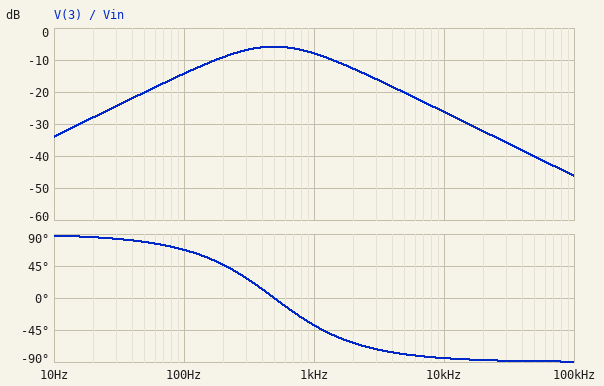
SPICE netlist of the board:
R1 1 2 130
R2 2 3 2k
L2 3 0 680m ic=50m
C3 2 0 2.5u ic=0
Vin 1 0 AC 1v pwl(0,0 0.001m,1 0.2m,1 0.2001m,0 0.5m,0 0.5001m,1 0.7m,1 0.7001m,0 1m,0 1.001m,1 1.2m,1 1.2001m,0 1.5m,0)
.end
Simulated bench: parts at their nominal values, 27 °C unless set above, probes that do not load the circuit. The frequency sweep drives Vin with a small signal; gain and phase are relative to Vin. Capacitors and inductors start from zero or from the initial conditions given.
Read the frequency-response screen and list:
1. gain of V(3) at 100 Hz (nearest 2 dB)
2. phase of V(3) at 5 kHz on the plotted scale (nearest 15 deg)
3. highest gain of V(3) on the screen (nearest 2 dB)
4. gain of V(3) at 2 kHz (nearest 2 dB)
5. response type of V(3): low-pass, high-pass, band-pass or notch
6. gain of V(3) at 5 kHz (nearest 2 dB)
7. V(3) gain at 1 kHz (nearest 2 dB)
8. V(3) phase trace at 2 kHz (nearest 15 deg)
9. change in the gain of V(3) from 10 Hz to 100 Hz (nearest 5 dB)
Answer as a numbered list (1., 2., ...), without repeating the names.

1. -14 dB
2. -75 deg
3. -6 dB
4. -12 dB
5. band-pass
6. -20 dB
7. -8 dB
8. -60 deg
9. 20 dB
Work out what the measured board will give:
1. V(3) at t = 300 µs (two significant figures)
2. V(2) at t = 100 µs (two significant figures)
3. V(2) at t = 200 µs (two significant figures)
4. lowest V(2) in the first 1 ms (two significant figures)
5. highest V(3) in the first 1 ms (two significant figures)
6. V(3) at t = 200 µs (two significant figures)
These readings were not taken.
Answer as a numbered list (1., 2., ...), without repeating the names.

1. -43 V
2. -1.2 V
3. -1.7 V
4. -2.1 V
5. -4.9 V
6. -57 V
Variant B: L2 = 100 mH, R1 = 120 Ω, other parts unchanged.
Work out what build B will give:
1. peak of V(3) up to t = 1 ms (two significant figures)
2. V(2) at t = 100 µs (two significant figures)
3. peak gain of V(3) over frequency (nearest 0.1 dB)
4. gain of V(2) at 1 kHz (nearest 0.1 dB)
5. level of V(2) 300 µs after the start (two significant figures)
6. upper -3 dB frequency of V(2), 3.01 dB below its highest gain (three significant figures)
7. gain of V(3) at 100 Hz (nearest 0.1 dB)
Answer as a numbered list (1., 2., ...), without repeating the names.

1. 120 mV
2. -410 mV
3. -16.9 dB
4. -6.6 dB
5. -82 mV
6. 569 Hz
7. -30.7 dB
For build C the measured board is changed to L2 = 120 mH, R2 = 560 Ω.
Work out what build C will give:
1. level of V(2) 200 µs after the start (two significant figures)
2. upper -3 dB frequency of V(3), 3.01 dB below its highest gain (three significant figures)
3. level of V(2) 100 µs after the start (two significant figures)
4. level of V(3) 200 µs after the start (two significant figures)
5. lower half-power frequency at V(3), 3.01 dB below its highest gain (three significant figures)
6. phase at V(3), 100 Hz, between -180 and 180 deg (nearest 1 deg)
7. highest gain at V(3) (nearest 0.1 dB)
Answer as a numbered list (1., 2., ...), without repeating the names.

1. -1.4 V
2. 1.53 kHz
3. -1.1 V
4. -12 V
5. 294 Hz
6. 74 deg
7. -8.0 dB
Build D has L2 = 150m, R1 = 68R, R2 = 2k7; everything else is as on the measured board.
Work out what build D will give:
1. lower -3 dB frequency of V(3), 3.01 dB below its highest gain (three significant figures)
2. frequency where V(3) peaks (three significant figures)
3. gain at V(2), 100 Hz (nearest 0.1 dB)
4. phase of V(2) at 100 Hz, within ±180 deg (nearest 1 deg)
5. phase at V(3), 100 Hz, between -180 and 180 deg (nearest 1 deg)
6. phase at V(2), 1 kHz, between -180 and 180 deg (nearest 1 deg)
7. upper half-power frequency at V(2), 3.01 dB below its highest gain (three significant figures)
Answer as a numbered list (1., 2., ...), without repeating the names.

1. 622 Hz
2. 1.66 kHz
3. -0.3 dB
4. -6 deg
5. 82 deg
6. -46 deg
7. 969 Hz
